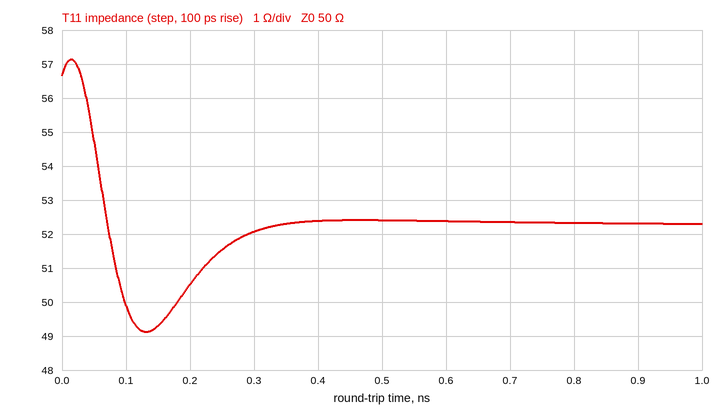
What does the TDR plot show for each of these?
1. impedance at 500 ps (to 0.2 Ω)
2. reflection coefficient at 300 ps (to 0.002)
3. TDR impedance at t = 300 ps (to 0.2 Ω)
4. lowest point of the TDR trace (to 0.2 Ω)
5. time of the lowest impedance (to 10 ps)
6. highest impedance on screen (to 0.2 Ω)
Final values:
52.4 Ω
+0.020
52.0 Ω
49.2 Ω
130 ps
57.2 Ω
